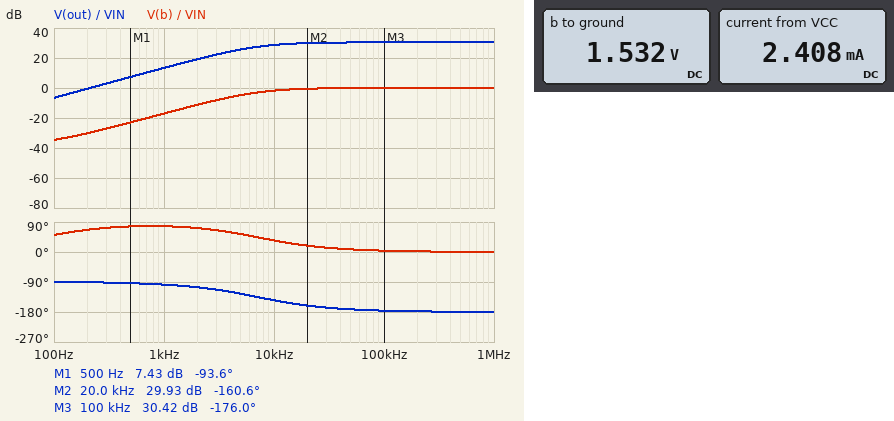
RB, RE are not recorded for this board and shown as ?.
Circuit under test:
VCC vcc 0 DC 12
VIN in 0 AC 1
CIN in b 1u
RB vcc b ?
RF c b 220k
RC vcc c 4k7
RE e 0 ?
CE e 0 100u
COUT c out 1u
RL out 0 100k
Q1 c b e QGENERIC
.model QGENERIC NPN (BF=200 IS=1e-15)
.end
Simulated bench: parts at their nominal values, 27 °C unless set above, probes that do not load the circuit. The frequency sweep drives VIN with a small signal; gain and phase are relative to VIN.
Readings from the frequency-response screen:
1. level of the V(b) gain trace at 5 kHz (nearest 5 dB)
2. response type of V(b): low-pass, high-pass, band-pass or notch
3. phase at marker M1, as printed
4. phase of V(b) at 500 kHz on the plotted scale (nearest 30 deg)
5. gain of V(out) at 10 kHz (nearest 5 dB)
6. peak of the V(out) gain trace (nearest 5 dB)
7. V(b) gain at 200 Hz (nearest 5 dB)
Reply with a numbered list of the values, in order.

1. -5 dB
2. high-pass
3. -93.6 deg
4. 0 deg
5. 30 dB
6. 30 dB
7. -30 dB
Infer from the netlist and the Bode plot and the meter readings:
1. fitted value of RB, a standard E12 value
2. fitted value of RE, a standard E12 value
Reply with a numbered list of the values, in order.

1. 220 kΩ
2. 330 Ω
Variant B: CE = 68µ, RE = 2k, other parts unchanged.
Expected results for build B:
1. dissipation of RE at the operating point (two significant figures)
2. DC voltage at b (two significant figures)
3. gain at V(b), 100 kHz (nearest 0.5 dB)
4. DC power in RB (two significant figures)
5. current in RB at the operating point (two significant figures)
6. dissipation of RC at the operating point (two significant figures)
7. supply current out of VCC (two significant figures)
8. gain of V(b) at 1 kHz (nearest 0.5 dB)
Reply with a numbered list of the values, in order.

1. 6.5 mW
2. 4.3 V
3. 0 dB
4. 270 µW
5. 35 µA
6. 15 mW
7. 1.8 mA
8. -14.5 dB
